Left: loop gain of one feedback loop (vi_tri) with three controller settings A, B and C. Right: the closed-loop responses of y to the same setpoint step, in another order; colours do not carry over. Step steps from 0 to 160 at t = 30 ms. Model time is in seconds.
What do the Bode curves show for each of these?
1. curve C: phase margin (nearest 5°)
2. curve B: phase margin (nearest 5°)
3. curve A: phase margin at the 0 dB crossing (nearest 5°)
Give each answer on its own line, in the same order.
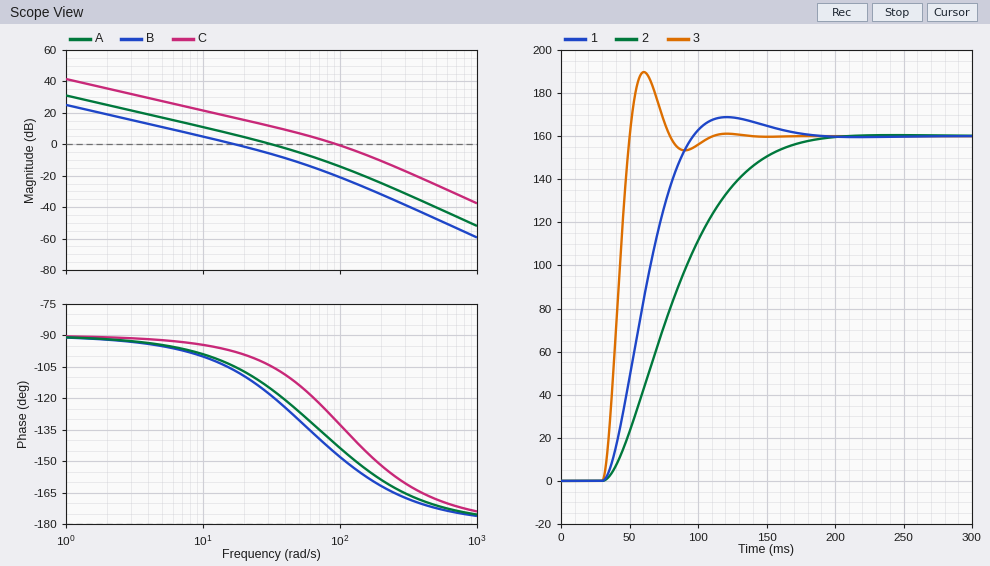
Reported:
50°
75°
65°
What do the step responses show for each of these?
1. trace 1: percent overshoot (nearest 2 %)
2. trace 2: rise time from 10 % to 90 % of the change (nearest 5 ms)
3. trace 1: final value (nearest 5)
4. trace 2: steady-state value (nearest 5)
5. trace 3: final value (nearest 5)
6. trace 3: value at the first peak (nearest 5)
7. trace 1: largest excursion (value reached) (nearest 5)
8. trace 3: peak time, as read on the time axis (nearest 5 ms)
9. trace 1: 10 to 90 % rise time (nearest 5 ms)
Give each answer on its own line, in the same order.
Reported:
6 %
90 ms
160
160
160
190
170
60 ms
45 ms
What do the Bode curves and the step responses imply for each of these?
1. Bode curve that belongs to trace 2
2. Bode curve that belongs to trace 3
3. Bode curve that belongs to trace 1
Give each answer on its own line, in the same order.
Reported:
B
C
A
